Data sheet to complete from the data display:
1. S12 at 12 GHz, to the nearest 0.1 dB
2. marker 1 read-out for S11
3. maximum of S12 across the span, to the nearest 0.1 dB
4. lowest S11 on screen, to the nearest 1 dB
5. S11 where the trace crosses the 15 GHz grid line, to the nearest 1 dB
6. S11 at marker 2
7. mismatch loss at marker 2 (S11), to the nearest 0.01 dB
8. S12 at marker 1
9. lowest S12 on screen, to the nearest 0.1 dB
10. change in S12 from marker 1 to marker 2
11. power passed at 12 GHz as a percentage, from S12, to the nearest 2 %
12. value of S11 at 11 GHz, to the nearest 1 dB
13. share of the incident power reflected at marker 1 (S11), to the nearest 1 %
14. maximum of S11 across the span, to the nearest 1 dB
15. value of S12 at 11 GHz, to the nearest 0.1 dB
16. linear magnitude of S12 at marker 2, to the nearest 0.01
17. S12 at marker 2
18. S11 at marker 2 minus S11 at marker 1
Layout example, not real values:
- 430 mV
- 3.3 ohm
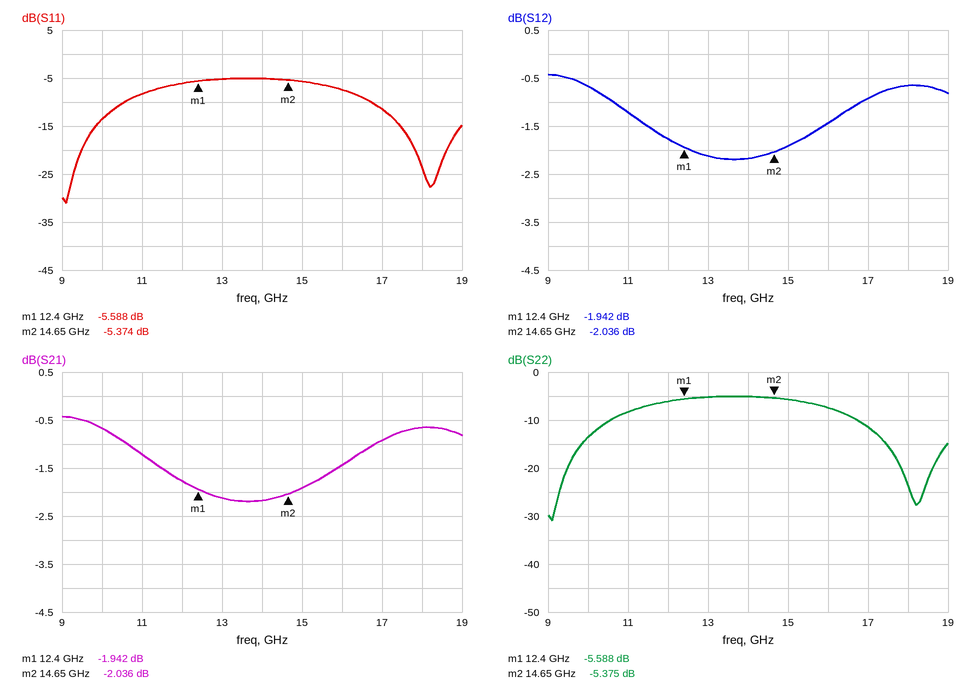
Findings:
- -1.8 dB
- -5.588 dB
- -0.4 dB
- -31 dB
- -6 dB
- -5.374 dB
- 1.49 dB
- -1.942 dB
- -2.2 dB
- -0.094 dB
- 66 %
- -8 dB
- 28 %
- -5 dB
- -1.2 dB
- 0.79
- -2.036 dB
- 0.214 dB
